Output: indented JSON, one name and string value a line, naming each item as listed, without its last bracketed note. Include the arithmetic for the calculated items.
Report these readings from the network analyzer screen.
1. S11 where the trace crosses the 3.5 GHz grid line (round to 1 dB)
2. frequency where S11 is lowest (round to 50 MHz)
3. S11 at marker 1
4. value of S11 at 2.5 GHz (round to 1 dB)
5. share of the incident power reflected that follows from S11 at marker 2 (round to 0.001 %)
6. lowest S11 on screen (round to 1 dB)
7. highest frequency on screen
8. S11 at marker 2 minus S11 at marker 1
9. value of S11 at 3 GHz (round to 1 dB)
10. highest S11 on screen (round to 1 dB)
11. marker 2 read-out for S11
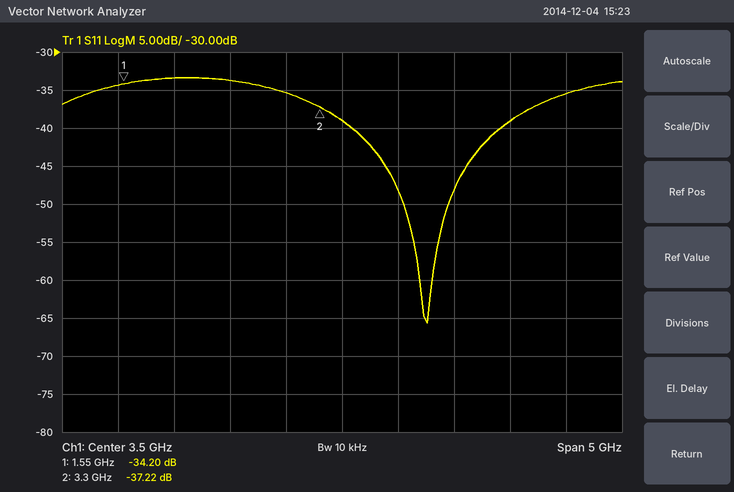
{
  "S11 where the trace crosses the 3.5 GHz grid line": "-39 dB",
  "frequency where S11 is lowest": "4.25 GHz",
  "S11 at marker 1": "-34.20 dB",
  "value of S11 at 2.5 GHz": "-34 dB",
  "share of the incident power reflected that follows from S11 at marker 2": "10^(-37.22/10) ≈ 0.019 %",
  "lowest S11 on screen": "-66 dB",
  "highest frequency on screen": "6 GHz",
  "S11 at marker 2 minus S11 at marker 1": "-37.22 − (-34.2) = -3.02 dB",
  "value of S11 at 3 GHz": "-35 dB",
  "highest S11 on screen": "-33 dB",
  "marker 2 read-out for S11": "-37.22 dB"
}
